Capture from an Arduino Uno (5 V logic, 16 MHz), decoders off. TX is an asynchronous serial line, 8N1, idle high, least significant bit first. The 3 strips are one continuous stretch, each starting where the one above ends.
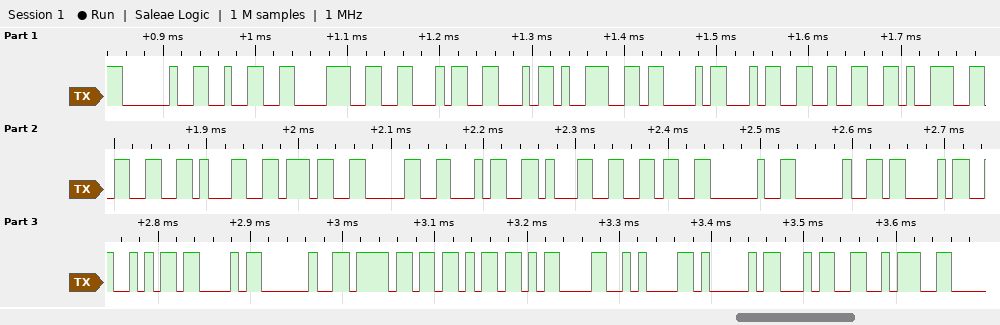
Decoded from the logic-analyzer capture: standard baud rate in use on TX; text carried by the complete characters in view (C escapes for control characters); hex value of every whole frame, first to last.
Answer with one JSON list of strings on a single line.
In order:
["115200 baud", "\" 28FF9C4293170416  CRC ok\\r\\nA4:\"", "0x20 0x32 0x38 0x46 0x46 0x39 0x43 0x34 0x32 0x39 0x33 0x31 0x37 0x30 0x34 0x31 0x36 0x20 0x20 0x43 0x52 0x43 0x20 0x6F 0x6B 0x0D 0x0A 0x41 0x34 0x3A"]
